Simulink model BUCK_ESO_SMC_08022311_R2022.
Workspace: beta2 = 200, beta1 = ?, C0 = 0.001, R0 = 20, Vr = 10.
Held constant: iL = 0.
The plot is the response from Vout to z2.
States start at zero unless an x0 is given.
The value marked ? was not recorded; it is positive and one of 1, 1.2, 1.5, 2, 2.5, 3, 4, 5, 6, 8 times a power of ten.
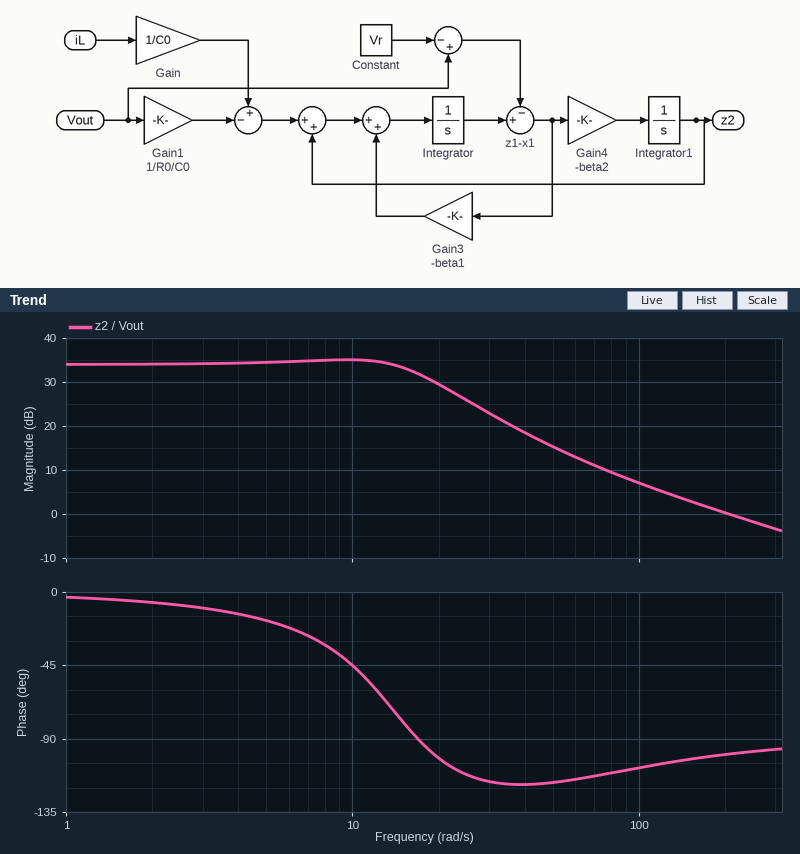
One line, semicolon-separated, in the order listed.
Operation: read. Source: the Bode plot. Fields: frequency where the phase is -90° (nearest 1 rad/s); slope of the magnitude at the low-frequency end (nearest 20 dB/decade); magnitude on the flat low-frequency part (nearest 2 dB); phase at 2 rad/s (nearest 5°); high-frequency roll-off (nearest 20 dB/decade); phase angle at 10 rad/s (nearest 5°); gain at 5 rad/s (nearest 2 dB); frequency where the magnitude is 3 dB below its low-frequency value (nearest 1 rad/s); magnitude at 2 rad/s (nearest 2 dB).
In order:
17 rad/s; 0 dB/decade; 34 dB; -5°; -20 dB/decade; -45°; 34 dB; 18 rad/s; 34 dB
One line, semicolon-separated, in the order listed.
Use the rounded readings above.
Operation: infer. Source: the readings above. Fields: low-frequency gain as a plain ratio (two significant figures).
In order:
50
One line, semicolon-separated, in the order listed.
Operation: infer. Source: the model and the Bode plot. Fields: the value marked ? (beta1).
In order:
15
